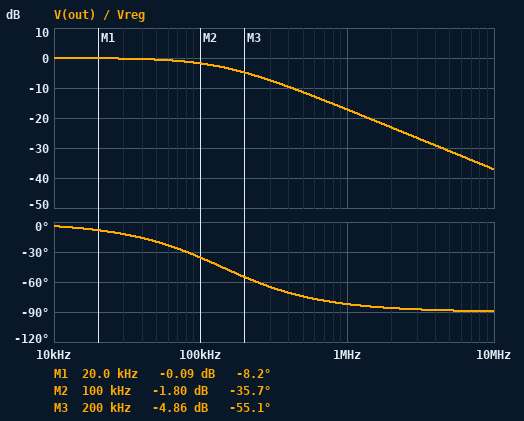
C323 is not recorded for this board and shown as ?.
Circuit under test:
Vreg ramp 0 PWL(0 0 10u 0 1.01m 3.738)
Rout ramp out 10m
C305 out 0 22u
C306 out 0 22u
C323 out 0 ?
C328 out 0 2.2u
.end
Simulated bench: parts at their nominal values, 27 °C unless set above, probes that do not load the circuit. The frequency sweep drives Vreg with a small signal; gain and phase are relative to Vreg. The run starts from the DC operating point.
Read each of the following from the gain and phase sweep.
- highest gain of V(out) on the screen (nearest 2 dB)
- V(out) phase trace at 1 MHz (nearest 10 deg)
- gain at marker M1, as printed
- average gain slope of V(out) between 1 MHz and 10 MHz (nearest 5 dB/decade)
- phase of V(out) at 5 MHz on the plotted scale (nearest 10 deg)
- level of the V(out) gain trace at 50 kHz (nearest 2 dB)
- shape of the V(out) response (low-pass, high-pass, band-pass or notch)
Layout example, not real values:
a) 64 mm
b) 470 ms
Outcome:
a) 0 dB
b) -80 deg
c) -0.09 dB
d) -20 dB/decade
e) -90 deg
f) 0 dB
g) low-pass
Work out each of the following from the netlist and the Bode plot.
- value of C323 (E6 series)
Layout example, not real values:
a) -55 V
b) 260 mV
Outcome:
a) 68 µF
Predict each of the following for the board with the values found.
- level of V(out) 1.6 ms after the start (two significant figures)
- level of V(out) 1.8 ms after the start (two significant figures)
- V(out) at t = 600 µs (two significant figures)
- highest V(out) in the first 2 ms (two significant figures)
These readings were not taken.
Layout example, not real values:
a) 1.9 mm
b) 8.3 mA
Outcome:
a) 3.7 V
b) 3.7 V
c) 2.2 V
d) 3.7 V
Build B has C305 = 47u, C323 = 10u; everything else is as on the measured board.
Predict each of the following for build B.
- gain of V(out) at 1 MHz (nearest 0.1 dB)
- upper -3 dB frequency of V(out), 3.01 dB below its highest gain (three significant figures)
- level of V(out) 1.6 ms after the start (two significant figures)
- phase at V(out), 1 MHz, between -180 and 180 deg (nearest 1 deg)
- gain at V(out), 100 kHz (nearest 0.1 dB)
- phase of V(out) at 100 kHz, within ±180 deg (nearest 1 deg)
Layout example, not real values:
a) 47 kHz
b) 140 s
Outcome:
a) -14.3 dB
b) 196 kHz
c) 3.7 V
d) -79 deg
e) -1.0 dB
f) -27 deg
